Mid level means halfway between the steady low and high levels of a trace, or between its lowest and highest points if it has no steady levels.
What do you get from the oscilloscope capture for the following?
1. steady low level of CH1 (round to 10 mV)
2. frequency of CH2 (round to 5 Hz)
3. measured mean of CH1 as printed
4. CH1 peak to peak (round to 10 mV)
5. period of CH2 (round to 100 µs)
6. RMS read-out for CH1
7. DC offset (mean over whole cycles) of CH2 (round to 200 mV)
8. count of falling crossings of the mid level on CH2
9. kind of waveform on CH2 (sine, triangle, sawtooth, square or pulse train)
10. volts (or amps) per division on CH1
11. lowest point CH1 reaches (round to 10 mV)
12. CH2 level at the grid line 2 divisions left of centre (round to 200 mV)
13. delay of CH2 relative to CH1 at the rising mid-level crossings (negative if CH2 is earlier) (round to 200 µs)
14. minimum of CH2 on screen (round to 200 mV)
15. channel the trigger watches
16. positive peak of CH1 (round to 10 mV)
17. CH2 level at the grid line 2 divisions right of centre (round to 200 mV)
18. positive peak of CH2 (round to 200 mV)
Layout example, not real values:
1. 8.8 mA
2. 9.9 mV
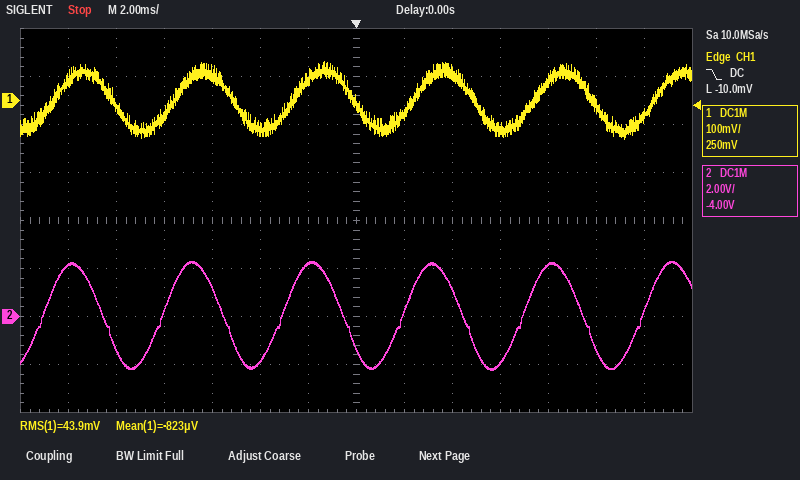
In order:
1. -60 mV
2. 200 Hz
3. -823 µV
4. 160 mV
5. 5.0 ms
6. 43.9 mV
7. 0.0 V
8. 5
9. sine
10. 100 mV
11. -80 mV
12. -1.8 V
13. -400 µs
14. -2.2 V
15. CH1
16. 80 mV
17. 1.2 V
18. 2.2 V
